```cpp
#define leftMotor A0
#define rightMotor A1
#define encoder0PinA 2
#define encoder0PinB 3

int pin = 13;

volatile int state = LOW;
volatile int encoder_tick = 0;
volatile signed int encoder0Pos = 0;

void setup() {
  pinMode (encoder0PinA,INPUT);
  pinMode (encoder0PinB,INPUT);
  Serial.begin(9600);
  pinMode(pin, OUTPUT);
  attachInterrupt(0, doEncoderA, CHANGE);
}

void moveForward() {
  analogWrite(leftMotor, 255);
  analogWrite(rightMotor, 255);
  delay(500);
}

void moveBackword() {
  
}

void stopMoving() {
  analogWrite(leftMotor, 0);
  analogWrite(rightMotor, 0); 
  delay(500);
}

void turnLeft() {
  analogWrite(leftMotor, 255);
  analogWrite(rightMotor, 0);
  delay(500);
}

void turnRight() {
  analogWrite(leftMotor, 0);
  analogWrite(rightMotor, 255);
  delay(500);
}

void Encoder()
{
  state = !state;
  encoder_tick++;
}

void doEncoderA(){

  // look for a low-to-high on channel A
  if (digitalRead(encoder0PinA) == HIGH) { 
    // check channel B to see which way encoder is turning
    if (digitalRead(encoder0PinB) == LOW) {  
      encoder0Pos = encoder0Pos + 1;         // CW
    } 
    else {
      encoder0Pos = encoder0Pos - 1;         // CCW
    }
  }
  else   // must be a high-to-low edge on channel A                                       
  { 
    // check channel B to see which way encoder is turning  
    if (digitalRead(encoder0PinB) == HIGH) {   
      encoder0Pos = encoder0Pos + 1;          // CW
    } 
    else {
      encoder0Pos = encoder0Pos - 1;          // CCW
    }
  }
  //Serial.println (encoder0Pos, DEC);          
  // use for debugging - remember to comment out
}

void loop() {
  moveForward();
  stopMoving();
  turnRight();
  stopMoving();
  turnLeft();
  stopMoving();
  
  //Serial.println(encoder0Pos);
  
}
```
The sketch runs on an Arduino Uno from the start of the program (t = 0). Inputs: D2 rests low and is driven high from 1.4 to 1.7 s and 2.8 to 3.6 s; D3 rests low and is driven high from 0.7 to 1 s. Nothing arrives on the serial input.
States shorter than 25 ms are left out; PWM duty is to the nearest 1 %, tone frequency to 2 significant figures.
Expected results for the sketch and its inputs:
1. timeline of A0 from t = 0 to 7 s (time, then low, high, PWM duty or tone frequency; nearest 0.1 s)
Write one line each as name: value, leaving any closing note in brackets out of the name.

timeline of A0 from t = 0 to 7 s: 0 s high; 0.5 s low; 2 s high; 2.5 s low; 3 s high; 3.5 s low; 5 s high; 5.5 s low; 6 s high; 6.5 s low
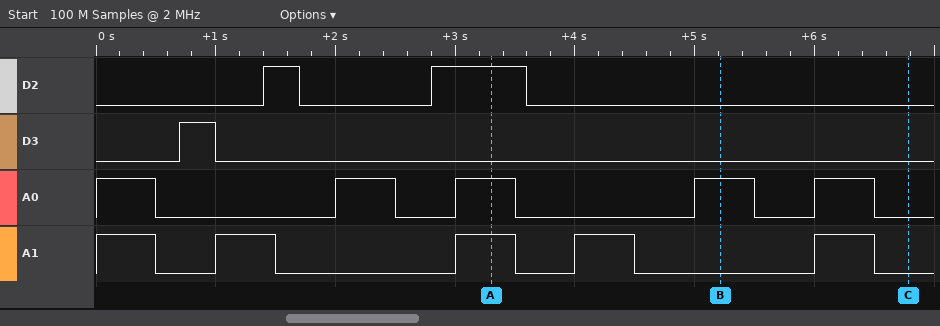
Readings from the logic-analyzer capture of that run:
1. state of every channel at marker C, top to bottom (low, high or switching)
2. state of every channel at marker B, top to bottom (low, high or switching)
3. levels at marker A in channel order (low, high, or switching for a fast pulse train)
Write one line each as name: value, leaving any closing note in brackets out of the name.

state of every channel at marker C, top to bottom: D2 low, D3 low, A0 low, A1 low
state of every channel at marker B, top to bottom: D2 low, D3 low, A0 high, A1 low
levels at marker A in channel order: D2 high, D3 low, A0 high, A1 high
